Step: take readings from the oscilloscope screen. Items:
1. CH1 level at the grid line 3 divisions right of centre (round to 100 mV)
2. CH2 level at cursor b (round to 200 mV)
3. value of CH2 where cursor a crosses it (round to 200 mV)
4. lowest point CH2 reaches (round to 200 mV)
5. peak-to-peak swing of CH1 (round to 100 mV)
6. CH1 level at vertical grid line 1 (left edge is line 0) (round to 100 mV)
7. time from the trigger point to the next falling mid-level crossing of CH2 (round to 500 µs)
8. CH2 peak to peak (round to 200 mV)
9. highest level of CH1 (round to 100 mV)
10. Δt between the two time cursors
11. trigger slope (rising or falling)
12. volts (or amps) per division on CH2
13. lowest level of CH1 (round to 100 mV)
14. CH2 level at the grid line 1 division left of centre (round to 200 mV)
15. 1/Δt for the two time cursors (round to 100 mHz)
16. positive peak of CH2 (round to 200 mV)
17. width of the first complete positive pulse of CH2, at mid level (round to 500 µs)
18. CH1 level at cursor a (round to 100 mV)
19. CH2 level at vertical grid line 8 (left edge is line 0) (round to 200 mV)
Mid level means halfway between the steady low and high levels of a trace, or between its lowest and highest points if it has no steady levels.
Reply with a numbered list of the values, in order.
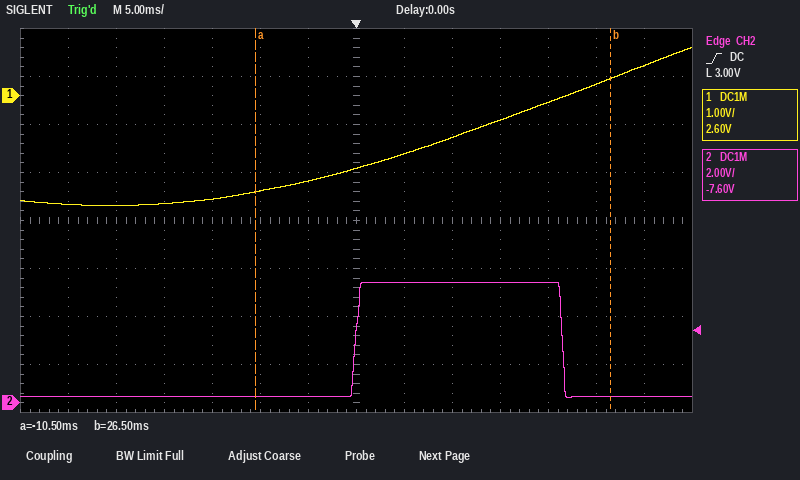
1. -500 mV
2. 200 mV
3. 200 mV
4. 200 mV
5. 3.3 V
6. -2.3 V
7. 21.5 ms
8. 4.8 V
9. 1.0 V
10. 37.0 ms
11. rising
12. 2 V
13. -2.3 V
14. 200 mV
15. 27.0 Hz
16. 5.0 V
17. 21.5 ms
18. -2.0 V
19. 5.0 V
